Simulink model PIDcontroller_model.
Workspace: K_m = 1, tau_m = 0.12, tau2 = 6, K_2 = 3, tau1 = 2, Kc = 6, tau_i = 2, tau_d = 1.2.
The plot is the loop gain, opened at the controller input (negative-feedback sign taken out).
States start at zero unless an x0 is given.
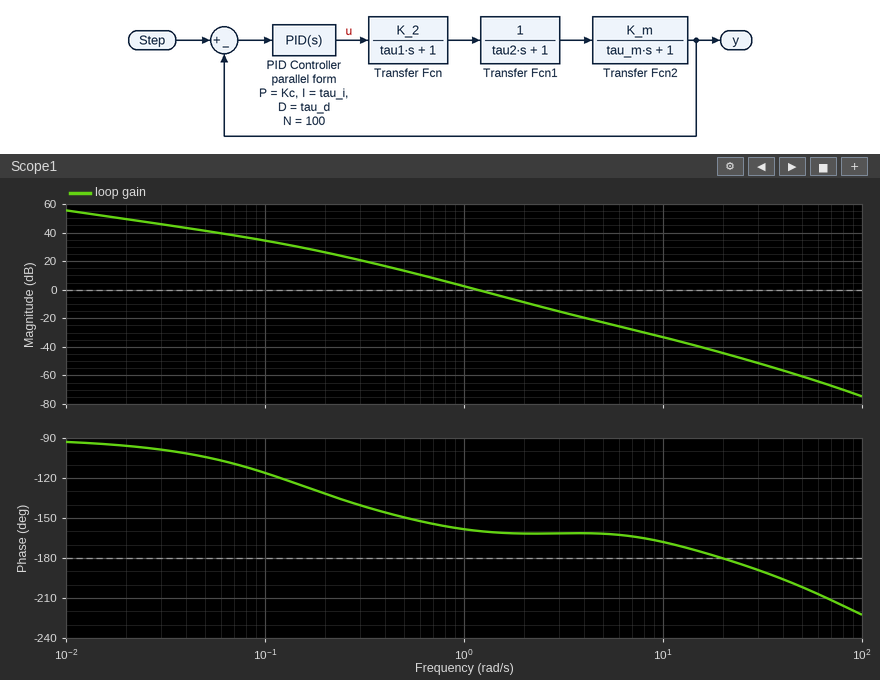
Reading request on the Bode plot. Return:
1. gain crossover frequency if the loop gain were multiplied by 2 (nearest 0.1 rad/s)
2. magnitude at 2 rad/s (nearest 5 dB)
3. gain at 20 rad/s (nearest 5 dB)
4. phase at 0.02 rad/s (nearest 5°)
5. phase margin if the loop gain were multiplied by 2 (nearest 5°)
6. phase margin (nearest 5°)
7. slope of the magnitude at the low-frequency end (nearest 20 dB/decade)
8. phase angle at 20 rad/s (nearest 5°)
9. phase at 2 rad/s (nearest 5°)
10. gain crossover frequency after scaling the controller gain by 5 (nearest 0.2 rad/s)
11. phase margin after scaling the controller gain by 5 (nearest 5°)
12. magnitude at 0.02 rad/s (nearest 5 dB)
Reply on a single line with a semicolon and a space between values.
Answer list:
1.7 rad/s; -10 dB; -45 dB; -95°; 20°; 20°; -20 dB/decade; -180°; -160°; 2.8 rad/s; 20°; 50 dB
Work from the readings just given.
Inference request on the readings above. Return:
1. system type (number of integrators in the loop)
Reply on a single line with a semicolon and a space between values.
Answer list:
1
